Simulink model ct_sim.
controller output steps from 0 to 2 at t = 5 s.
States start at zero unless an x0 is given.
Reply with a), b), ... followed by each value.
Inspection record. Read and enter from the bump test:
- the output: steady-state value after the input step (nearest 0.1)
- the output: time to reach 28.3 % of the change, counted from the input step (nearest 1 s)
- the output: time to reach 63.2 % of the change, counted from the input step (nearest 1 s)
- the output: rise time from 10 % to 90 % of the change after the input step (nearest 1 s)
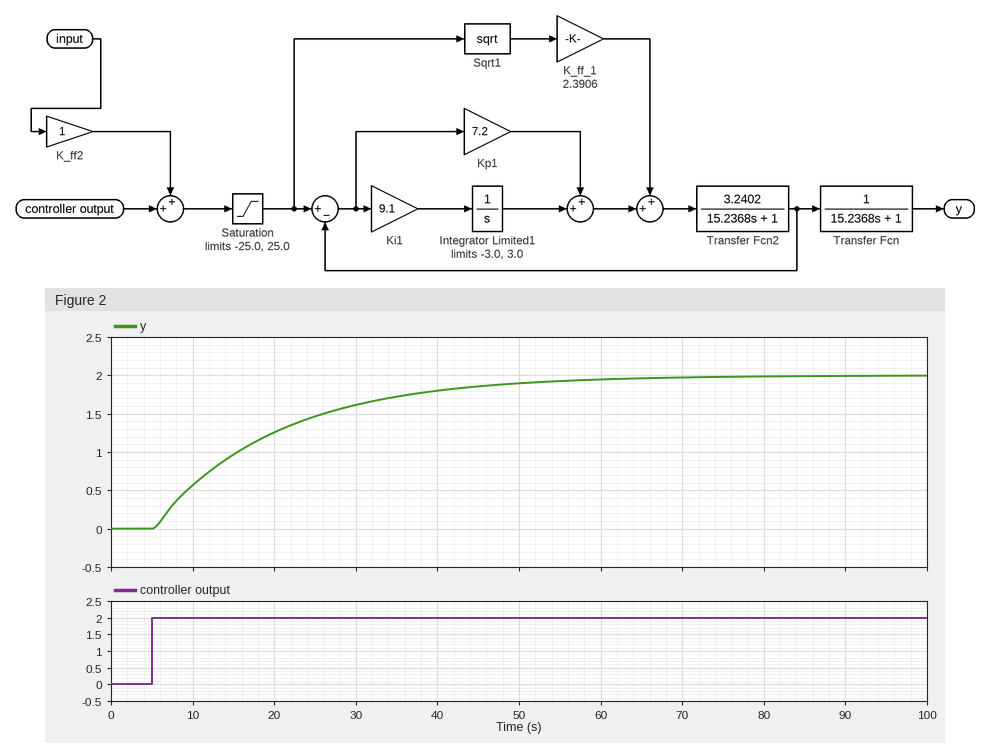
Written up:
a) 2.0
b) 5 s
c) 15 s
d) 33 s
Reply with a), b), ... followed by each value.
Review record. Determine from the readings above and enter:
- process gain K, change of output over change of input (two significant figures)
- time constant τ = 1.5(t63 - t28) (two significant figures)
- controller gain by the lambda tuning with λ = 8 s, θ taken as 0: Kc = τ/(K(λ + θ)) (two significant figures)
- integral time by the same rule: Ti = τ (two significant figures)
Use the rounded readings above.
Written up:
a) 1.0
b) 15 s
c) 1.9
d) 15 s
